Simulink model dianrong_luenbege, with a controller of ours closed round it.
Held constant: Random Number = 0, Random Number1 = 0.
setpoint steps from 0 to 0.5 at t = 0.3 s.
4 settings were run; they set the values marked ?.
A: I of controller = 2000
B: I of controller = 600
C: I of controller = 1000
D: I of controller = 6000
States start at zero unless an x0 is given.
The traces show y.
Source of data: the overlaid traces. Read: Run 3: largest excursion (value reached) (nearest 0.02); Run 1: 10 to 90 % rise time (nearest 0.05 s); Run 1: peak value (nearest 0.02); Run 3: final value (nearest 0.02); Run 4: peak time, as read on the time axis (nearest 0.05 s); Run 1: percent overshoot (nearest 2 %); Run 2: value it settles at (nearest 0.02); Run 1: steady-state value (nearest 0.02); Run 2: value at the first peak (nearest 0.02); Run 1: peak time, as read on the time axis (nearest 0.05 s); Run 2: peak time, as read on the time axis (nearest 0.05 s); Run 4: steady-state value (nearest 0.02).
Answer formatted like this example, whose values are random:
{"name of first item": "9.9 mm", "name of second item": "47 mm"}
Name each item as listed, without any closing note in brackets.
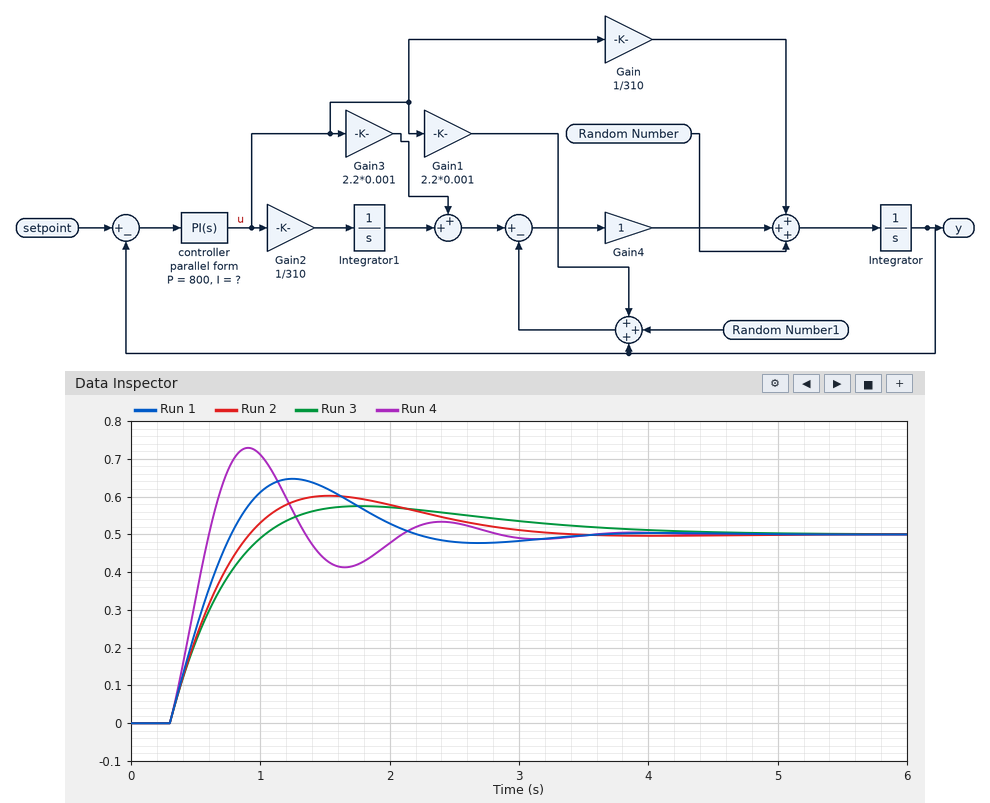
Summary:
{"Run 3: largest excursion (value reached)": "0.58", "Run 1: 10 to 90 % rise time": "0.35 s", "Run 1: peak value": "0.64", "Run 3: final value": "0.50", "Run 4: peak time, as read on the time axis": "0.90 s", "Run 1: percent overshoot": "30 %", "Run 2: value it settles at": "0.50", "Run 1: steady-state value": "0.50", "Run 2: value at the first peak": "0.60", "Run 1: peak time, as read on the time axis": "1.25 s", "Run 2: peak time, as read on the time axis": "1.55 s", "Run 4: steady-state value": "0.50"}
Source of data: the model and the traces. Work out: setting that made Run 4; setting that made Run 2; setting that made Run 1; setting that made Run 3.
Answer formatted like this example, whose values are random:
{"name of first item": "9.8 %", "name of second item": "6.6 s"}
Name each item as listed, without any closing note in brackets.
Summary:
{"setting that made Run 4": "D", "setting that made Run 2": "C", "setting that made Run 1": "A", "setting that made Run 3": "B"}
